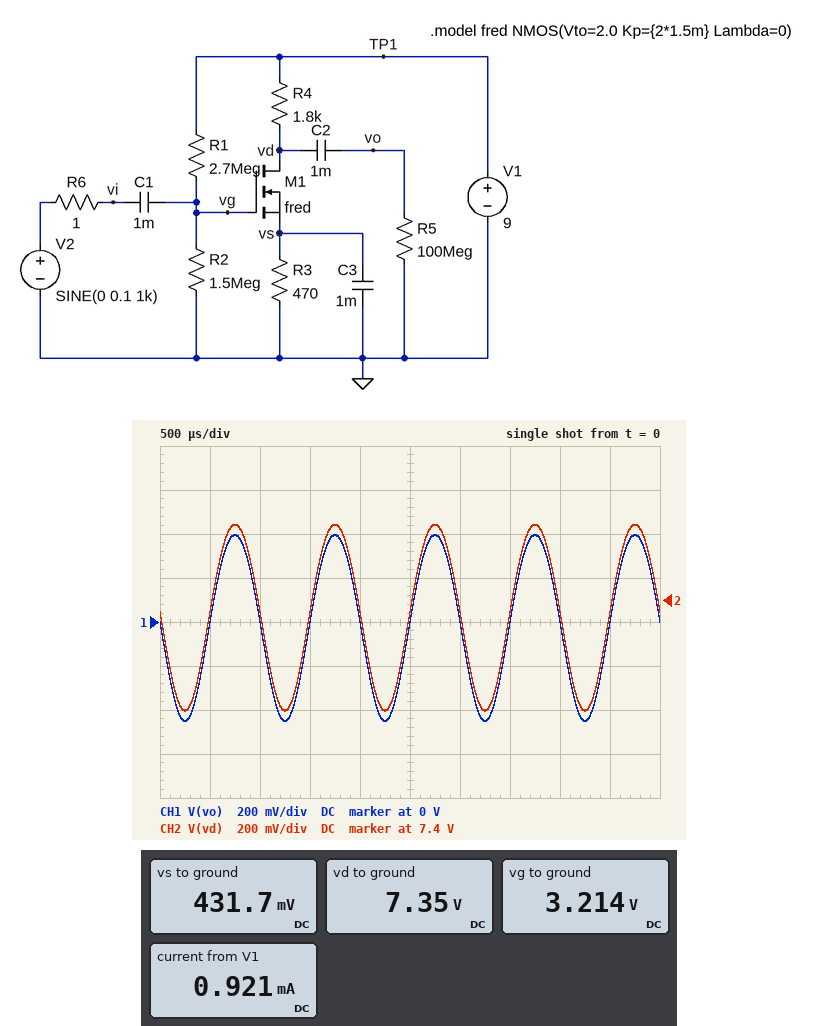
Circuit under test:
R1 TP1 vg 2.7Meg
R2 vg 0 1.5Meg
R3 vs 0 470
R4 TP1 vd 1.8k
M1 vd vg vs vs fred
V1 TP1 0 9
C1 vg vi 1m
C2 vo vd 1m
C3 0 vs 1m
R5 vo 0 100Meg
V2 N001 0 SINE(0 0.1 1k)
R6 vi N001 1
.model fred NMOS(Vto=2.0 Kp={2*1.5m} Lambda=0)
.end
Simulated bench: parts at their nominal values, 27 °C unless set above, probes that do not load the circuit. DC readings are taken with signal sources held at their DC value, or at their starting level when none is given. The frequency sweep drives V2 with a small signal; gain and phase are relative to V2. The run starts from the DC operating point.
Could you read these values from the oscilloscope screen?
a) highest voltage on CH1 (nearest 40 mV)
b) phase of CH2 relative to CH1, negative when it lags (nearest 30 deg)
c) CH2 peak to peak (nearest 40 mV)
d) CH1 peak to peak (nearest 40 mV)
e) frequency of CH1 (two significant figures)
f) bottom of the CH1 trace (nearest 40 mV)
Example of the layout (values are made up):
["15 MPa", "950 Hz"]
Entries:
["400 mV", "0 deg", "840 mV", "840 mV", "1.0 kHz", "-440 mV"]
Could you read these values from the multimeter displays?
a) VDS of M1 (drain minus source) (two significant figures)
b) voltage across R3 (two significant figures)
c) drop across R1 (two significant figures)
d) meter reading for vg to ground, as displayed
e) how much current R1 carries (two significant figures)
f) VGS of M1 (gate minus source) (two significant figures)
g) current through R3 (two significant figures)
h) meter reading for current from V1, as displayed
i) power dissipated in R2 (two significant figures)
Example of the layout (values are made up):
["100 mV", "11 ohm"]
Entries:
["6.9 V", "430 mV", "5.8 V", "3.214 V", "2.1 µA", "2.8 V", "920 µA", "0.921 mA", "6.9 µW"]
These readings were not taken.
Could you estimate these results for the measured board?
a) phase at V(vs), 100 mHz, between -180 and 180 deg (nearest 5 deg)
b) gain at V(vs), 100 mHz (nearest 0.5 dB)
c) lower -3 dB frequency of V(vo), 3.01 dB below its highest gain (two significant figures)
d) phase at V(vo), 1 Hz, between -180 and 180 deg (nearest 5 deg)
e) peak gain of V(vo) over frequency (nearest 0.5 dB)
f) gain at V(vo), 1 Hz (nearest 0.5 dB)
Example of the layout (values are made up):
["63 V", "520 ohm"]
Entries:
["-10 deg", "-5.5 dB", "530 mHz", "-165 deg", "12.5 dB", "11.0 dB"]
